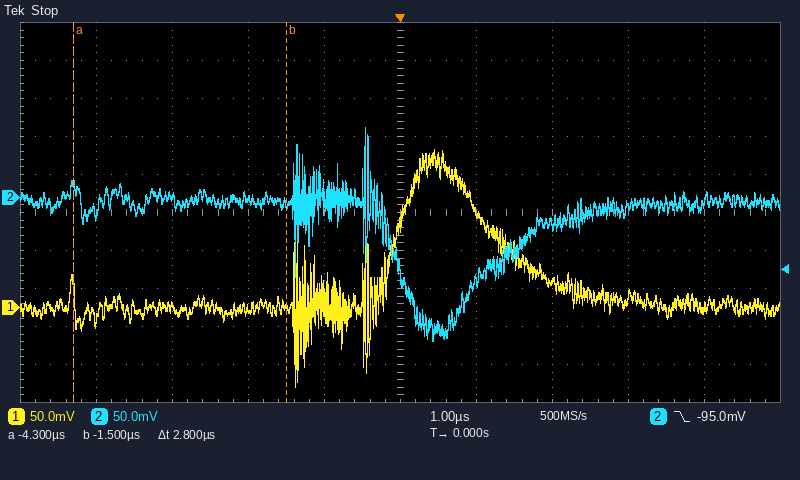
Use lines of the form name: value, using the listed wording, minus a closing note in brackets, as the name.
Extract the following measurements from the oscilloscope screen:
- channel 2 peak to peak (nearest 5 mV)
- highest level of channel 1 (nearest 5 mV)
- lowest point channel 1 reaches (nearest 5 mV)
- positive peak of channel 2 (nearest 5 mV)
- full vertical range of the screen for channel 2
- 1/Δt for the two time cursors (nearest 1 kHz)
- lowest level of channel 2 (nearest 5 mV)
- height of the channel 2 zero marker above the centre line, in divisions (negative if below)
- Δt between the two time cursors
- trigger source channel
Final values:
channel 2 peak to peak: 280 mV
highest level of channel 1: 210 mV
lowest point channel 1 reaches: -105 mV
positive peak of channel 2: 90 mV
full vertical range of the screen for channel 2: 500 mV
1/Δt for the two time cursors: 357 kHz
lowest level of channel 2: -190 mV
height of the channel 2 zero marker above the centre line, in divisions: +0.4 div
Δt between the two time cursors: 2.8 µs
trigger source channel: channel 2
